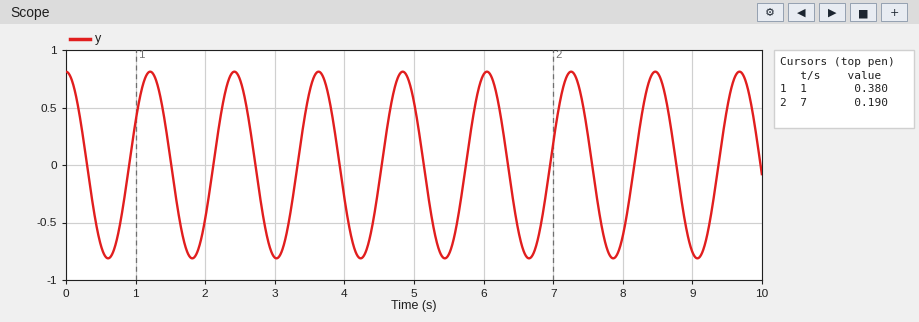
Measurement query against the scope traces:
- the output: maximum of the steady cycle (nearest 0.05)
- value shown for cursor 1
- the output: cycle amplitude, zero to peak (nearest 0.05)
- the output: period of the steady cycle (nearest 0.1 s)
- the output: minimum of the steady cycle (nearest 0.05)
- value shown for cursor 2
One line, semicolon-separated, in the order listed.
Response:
0.80; 0.380; 0.80; 1.2 s; -0.80; 0.190
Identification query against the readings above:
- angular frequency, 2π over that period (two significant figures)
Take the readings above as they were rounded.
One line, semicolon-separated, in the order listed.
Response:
5.2 rad/s
